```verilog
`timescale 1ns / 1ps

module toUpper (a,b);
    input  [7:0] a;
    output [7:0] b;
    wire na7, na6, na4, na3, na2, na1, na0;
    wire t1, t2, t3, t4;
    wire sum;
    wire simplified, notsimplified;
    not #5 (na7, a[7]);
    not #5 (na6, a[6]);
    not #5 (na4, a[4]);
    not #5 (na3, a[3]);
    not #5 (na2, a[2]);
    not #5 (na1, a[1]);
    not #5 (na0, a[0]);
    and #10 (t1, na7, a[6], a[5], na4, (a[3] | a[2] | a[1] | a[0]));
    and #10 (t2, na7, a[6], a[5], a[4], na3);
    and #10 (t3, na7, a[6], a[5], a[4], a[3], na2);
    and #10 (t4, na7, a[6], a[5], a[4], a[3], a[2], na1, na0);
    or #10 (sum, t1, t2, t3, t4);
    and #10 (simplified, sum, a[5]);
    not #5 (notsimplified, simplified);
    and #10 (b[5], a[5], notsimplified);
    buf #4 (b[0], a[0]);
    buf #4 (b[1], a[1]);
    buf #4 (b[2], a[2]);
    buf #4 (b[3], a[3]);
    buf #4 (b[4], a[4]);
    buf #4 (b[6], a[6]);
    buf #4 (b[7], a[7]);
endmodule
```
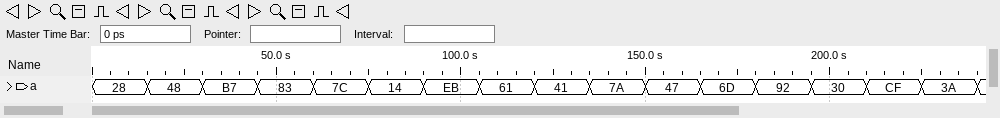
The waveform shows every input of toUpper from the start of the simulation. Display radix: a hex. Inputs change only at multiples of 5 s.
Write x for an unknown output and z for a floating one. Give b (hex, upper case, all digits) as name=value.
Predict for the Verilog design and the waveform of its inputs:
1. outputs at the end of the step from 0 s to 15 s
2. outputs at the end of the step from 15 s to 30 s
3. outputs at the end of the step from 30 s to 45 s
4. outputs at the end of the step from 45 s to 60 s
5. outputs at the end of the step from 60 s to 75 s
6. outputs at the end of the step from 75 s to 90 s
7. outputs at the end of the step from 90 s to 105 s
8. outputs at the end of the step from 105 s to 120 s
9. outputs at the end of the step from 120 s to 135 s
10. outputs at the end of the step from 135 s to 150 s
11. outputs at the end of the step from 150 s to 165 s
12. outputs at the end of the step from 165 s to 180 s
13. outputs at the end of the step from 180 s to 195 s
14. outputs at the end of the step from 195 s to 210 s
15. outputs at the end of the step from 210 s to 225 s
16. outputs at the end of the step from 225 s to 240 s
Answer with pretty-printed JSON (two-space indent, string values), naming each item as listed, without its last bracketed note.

{
  "outputs at the end of the step from 0 s to 15 s": "b=28",
  "outputs at the end of the step from 15 s to 30 s": "b=48",
  "outputs at the end of the step from 30 s to 45 s": "b=B7",
  "outputs at the end of the step from 45 s to 60 s": "b=83",
  "outputs at the end of the step from 60 s to 75 s": "b=5C",
  "outputs at the end of the step from 75 s to 90 s": "b=14",
  "outputs at the end of the step from 90 s to 105 s": "b=EB",
  "outputs at the end of the step from 105 s to 120 s": "b=41",
  "outputs at the end of the step from 120 s to 135 s": "b=41",
  "outputs at the end of the step from 135 s to 150 s": "b=5A",
  "outputs at the end of the step from 150 s to 165 s": "b=47",
  "outputs at the end of the step from 165 s to 180 s": "b=4D",
  "outputs at the end of the step from 180 s to 195 s": "b=92",
  "outputs at the end of the step from 195 s to 210 s": "b=30",
  "outputs at the end of the step from 210 s to 225 s": "b=CF",
  "outputs at the end of the step from 225 s to 240 s": "b=3A"
}
